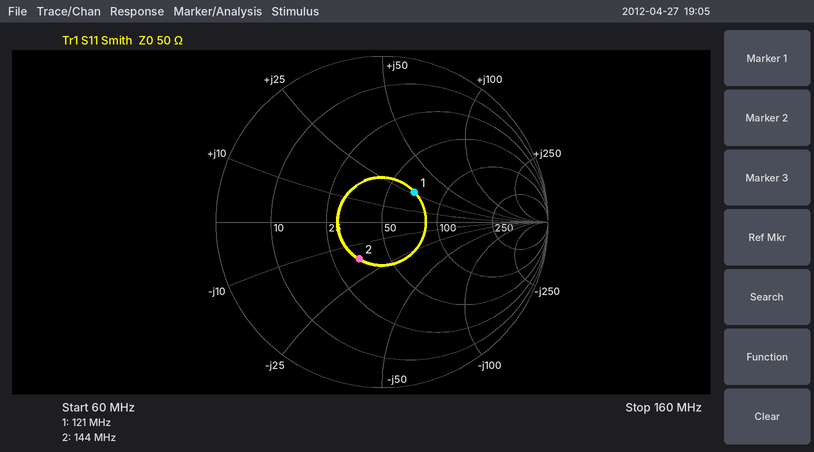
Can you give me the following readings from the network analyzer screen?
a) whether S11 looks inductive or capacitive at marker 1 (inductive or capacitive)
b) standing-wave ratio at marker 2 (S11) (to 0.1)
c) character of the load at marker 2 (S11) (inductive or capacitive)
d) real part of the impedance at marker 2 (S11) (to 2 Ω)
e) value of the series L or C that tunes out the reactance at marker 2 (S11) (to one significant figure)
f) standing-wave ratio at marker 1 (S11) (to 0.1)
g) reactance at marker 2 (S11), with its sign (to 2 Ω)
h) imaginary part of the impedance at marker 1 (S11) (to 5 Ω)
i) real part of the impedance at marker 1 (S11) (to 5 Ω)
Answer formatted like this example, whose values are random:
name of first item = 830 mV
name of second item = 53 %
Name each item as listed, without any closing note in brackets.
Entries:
whether S11 looks inductive or capacitive at marker 1 = inductive
standing-wave ratio at marker 2 (S11) = 1.7
character of the load at marker 2 (S11) = capacitive
real part of the impedance at marker 2 (S11) = 34 Ω
value of the series L or C that tunes out the reactance at marker 2 (S11) = 20 nH
standing-wave ratio at marker 1 (S11) = 1.7
reactance at marker 2 (S11), with its sign = -16 Ω
imaginary part of the impedance at marker 1 (S11) = +25 Ω
real part of the impedance at marker 1 (S11) = 70 Ω
